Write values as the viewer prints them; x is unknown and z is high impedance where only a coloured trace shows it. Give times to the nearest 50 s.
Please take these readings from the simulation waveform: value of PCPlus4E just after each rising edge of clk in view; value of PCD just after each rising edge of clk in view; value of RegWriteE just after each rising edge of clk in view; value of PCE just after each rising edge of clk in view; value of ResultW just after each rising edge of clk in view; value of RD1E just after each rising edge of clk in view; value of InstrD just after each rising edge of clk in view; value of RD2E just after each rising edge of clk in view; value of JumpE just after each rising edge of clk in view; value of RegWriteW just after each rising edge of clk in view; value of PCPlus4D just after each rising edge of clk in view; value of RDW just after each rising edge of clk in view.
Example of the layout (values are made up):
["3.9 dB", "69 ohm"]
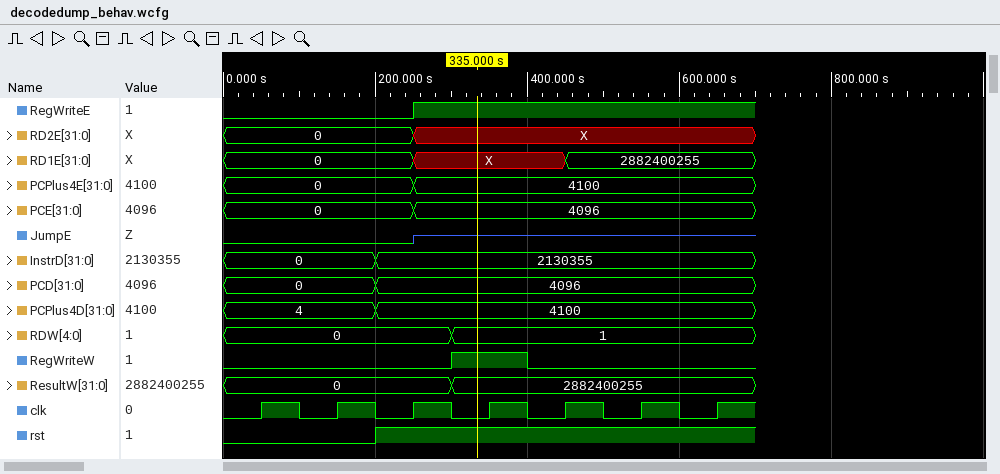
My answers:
["0, 0, 4100, 4100, 4100, 4100, 4100", "0, 0, 4096, 4096, 4096, 4096, 4096", "0 0 1 1 1 1 1", "0, 0, 4096, 4096, 4096, 4096, 4096", "0, 0, 0, 2882400255, 2882400255, 2882400255, 2882400255", "0, 0, X, X, 2882400255, 2882400255, 2882400255", "0, 0, 2130355, 2130355, 2130355, 2130355, 2130355", "0, 0, X, X, X, X, X", "0 0 z z z z z", "0 0 0 1 0 0 0", "4, 4, 4100, 4100, 4100, 4100, 4100", "0, 0, 0, 1, 1, 1, 1"]
